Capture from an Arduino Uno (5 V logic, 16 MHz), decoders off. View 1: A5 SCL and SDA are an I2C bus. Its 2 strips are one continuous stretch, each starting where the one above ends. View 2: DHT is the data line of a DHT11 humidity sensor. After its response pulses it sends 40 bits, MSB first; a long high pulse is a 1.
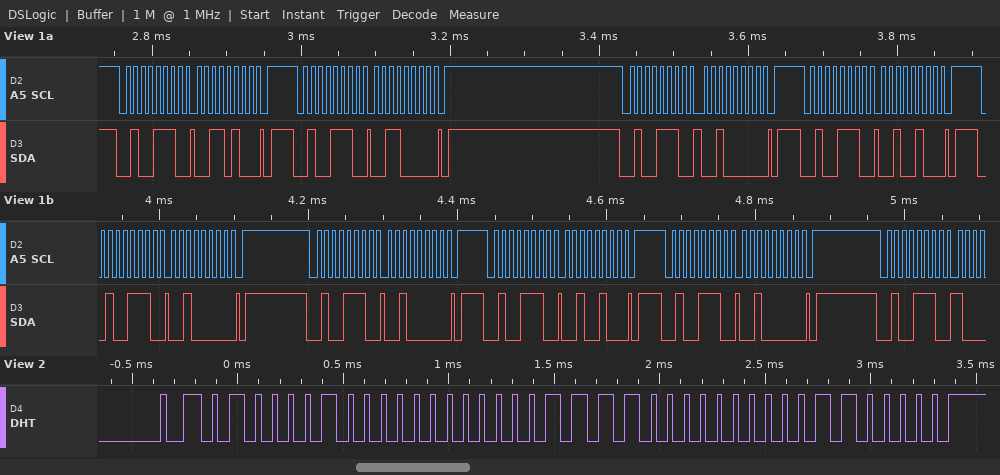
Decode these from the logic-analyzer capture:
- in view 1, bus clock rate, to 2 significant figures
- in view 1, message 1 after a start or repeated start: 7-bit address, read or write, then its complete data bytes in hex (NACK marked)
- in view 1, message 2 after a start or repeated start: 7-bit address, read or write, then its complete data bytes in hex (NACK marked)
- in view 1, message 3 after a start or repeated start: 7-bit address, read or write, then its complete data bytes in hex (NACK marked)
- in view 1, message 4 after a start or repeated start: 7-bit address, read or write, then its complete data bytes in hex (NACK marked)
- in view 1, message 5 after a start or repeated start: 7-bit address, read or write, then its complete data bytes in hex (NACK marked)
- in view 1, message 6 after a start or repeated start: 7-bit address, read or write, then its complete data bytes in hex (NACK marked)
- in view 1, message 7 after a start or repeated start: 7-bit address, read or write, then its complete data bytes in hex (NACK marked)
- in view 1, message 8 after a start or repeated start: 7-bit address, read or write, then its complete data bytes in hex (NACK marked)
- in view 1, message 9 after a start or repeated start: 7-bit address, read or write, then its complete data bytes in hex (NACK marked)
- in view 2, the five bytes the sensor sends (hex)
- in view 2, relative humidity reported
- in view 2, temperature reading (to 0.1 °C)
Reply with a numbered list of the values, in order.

1. 100 kHz
2. 0x27 write: 34
3. 0x27 write: 30
4. 0x27 write: 20
5. 0x27 write: 24
6. 0x27 write: 20
7. 0x27 write: 20
8. 0x27 write: 24
9. 0x27 write: 20
10. 0x27 write
11. 42 00 1E 00 60
12. 66 %
13. 30.0 °C
